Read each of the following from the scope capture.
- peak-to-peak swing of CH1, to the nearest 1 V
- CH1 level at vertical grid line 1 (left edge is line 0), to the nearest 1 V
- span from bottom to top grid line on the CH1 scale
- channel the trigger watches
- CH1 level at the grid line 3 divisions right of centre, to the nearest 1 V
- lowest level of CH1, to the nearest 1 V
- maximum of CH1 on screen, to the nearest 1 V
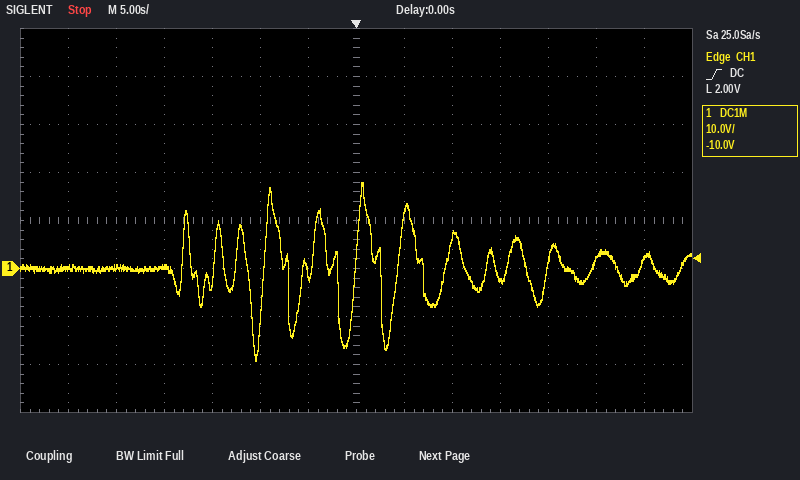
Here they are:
37 V
0 V
80 V
CH1
-2 V
-19 V
18 V
